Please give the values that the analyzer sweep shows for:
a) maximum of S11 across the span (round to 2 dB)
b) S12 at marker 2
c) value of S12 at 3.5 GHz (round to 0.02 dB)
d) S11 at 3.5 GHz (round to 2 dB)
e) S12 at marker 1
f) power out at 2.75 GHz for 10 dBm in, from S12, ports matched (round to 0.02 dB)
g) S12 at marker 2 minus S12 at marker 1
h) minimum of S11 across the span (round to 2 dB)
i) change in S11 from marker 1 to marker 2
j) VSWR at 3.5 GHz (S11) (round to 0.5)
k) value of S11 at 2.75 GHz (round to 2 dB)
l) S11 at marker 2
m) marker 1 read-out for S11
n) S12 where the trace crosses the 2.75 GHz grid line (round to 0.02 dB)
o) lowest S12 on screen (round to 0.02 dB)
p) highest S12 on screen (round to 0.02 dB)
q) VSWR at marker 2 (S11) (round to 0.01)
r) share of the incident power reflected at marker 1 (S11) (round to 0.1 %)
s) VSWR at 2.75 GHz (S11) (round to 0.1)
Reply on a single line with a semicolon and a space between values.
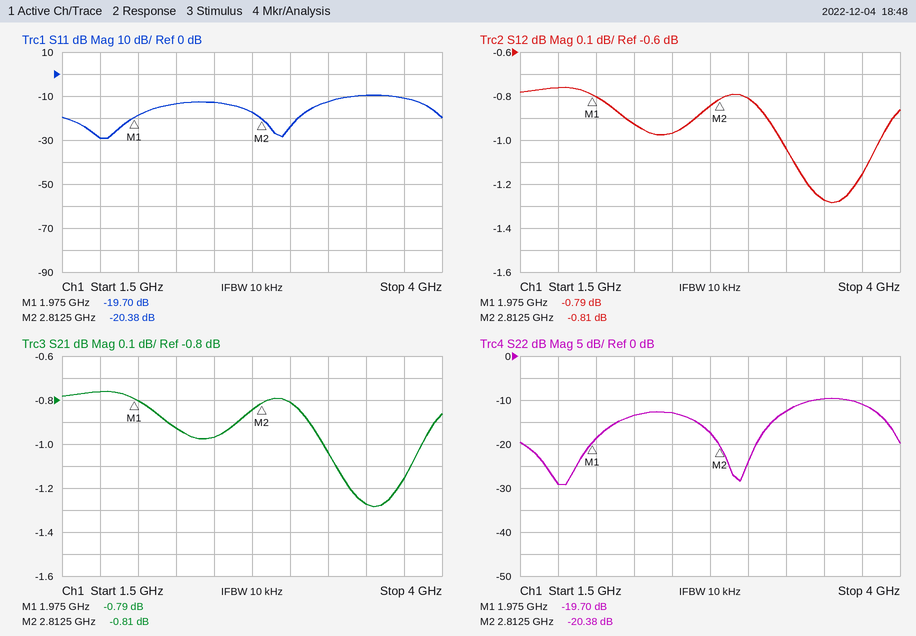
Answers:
-10 dB; -0.81 dB; -1.28 dB; -10 dB; -0.79 dB; 9.16 dBm; -0.02 dB; -30 dB; -0.68 dB; 2.0; -18 dB; -20.38 dB; -19.70 dB; -0.84 dB; -1.28 dB; -0.76 dB; 1.21; 1.1 %; 1.3
